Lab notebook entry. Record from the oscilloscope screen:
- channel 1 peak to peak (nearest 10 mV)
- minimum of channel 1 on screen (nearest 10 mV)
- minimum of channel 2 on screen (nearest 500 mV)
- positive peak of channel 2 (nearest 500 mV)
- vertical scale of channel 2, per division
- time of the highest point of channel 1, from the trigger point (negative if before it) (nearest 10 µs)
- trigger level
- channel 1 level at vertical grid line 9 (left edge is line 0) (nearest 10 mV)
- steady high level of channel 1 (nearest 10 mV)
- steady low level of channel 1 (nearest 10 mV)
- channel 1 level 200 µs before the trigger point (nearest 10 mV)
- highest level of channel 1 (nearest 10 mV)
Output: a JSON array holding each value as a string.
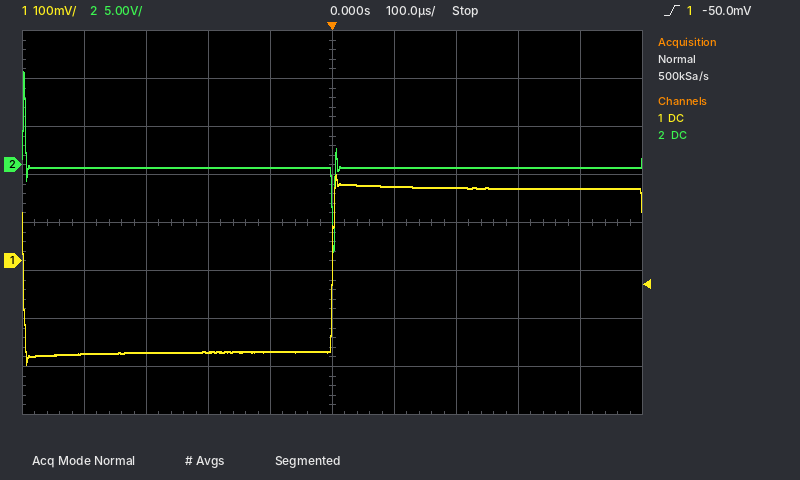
["400 mV", "-220 mV", "-9.0 V", "9.5 V", "5 V", "+10 µs", "-50.0 mV", "150 mV", "150 mV", "-190 mV", "-190 mV", "180 mV"]
